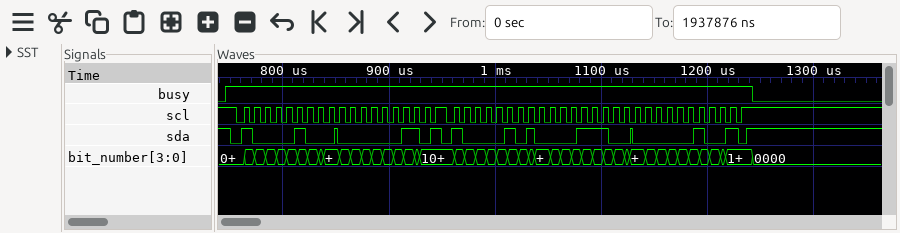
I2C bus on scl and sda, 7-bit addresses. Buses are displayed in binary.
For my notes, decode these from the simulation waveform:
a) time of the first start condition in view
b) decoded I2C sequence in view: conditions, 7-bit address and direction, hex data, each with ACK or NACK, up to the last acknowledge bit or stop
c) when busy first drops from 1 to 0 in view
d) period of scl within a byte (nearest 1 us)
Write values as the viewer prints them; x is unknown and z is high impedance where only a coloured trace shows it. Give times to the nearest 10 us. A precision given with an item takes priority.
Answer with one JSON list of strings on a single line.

["750 us", "start, address 42 write ACK, 03 ACK, repeated start, address 42 read ACK, 1C ACK, 04 NACK, stop", "1240 us", "10 us"]
